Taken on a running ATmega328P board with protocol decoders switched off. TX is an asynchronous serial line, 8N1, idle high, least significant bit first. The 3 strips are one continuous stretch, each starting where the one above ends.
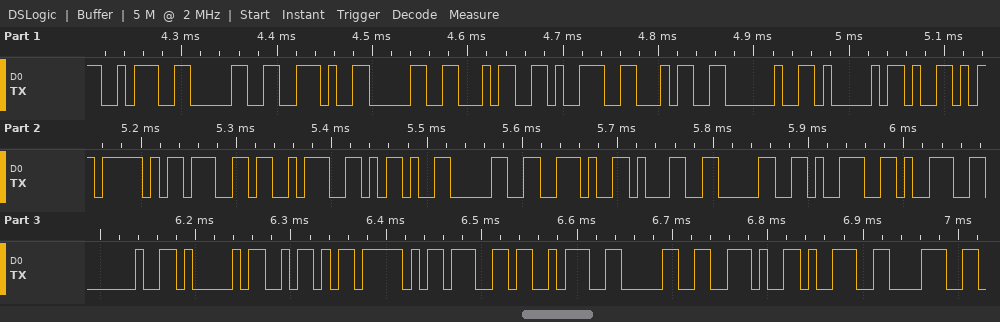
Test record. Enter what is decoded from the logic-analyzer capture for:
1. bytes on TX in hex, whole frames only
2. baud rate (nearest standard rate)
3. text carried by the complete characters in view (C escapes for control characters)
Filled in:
3A 30 2E 30 34 39 34 20 41 59 5F 67 3A 2D 30 2E 31 30 39 39 20 41 5A 5F 67 3A 30 2E 39 38
115200 baud
":0.0494 AY_g:-0.1099 AZ_g:0.98"
